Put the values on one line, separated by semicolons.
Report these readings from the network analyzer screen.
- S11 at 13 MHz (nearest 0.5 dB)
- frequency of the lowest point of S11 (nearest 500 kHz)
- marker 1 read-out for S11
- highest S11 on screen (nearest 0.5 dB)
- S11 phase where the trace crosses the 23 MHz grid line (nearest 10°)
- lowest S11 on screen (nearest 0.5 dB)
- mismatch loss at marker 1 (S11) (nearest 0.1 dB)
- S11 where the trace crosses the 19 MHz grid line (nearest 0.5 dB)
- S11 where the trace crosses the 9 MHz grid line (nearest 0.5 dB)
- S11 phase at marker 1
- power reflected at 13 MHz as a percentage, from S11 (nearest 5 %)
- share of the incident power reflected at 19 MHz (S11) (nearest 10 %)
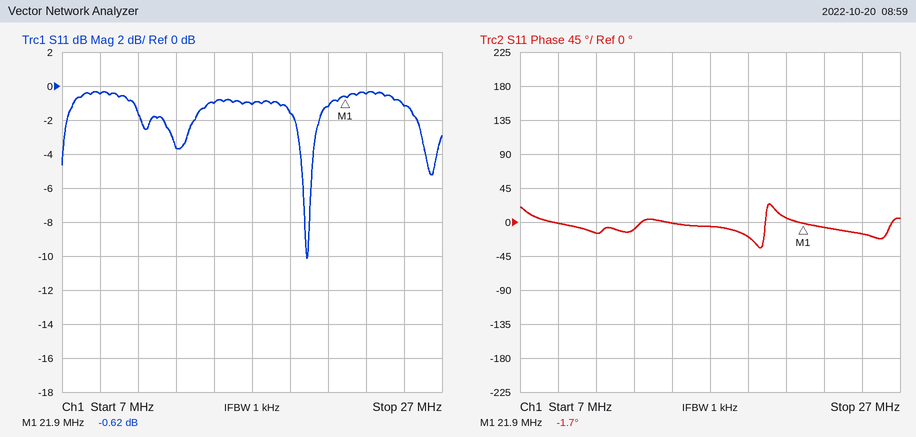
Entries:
-3.5 dB; 20.0 MHz; -0.62 dB; -0.5 dB; -10°; -10.0 dB; 8.8 dB; -1.5 dB; -0.5 dB; -1.7°; 45 %; 70 %
